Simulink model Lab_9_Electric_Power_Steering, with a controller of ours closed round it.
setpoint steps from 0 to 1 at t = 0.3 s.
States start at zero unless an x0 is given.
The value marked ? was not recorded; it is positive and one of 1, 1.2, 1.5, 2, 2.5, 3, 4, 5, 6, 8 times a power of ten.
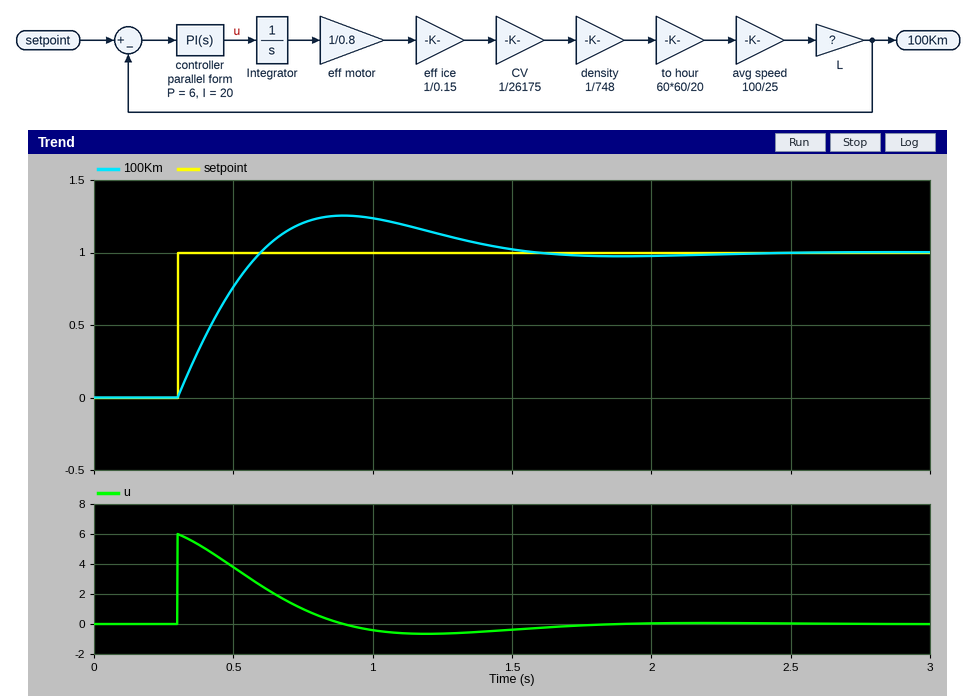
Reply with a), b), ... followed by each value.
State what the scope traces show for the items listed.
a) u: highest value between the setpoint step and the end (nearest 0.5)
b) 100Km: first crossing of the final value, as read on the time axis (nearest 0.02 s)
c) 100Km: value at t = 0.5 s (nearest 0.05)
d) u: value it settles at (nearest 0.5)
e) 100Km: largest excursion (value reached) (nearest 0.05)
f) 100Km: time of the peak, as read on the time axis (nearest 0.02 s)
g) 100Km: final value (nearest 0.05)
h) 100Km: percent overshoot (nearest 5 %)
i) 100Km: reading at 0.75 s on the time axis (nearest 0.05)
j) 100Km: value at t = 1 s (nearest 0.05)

a) 6.0
b) 0.60 s
c) 0.75
d) 0.0
e) 1.25
f) 0.90 s
g) 1.00
h) 25 %
i) 1.20
j) 1.25
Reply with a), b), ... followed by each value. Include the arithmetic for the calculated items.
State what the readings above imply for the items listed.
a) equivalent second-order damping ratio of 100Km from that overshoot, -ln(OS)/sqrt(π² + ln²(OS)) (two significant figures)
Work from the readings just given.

a) ln(0.25) = -1.386; 1.386 / sqrt(9.870 + 1.922) = 0.40
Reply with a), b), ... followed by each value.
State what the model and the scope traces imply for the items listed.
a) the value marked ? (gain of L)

a) 2500
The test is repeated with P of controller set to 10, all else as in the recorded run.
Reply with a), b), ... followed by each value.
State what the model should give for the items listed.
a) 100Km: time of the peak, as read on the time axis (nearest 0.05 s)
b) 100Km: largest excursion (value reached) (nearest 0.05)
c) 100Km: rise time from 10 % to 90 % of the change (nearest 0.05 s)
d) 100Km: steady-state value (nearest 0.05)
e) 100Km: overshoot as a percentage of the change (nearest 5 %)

a) 0.80 s
b) 1.15
c) 0.20 s
d) 1.00
e) 15 %
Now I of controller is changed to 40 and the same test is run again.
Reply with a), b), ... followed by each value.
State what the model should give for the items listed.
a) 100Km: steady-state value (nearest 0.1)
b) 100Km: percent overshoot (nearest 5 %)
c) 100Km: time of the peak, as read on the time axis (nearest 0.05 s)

a) 1.0
b) 35 %
c) 0.75 s
